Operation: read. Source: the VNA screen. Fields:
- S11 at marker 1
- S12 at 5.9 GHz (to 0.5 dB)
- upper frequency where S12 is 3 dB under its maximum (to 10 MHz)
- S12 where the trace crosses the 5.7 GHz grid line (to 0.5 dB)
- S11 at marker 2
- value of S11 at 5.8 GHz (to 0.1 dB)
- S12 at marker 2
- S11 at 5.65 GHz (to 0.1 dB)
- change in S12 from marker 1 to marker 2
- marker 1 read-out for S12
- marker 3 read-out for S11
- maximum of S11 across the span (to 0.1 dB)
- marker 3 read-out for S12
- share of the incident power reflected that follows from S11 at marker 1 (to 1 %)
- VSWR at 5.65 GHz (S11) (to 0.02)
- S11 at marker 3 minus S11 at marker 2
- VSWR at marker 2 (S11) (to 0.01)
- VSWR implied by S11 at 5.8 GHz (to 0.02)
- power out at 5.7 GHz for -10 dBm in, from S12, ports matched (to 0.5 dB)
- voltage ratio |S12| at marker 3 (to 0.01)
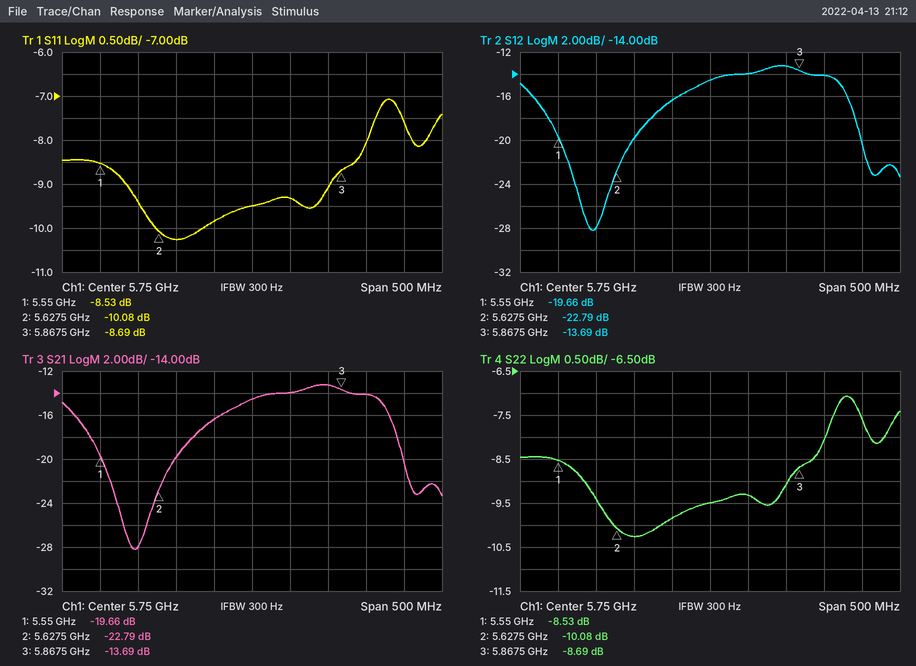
-8.53 dB
-14.0 dB
5.93 GHz
-16.5 dB
-10.08 dB
-9.3 dB
-22.79 dB
-10.3 dB
-3.13 dB
-19.66 dB
-8.69 dB
-7.1 dB
-13.69 dB
14 %
1.88
1.39 dB
1.91
2.04
-26.5 dBm
0.21
